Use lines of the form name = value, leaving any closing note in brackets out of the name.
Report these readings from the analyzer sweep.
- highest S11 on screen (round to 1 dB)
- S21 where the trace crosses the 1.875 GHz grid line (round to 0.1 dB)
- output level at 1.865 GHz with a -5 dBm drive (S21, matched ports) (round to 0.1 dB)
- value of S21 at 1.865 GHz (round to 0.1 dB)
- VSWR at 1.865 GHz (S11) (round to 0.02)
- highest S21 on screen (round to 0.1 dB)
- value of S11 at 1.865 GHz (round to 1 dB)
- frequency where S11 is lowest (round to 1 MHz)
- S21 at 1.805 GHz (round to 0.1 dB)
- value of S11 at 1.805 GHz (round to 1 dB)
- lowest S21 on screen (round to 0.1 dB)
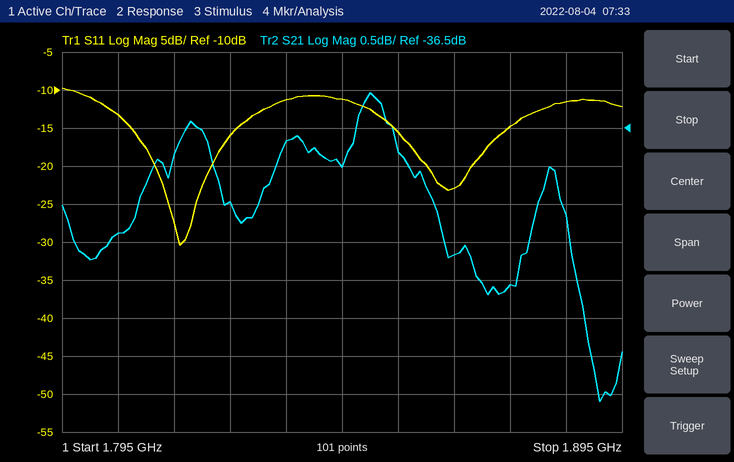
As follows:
highest S11 on screen = -10 dB
S21 where the trace crosses the 1.875 GHz grid line = -38.6 dB
output level at 1.865 GHz with a -5 dBm drive (S21, matched ports) = -43.2 dBm
value of S21 at 1.865 GHz = -38.2 dB
VSWR at 1.865 GHz (S11) = 1.16
highest S21 on screen = -36.0 dB
value of S11 at 1.865 GHz = -23 dB
frequency where S11 is lowest = 1.816 GHz
S21 at 1.805 GHz = -37.9 dB
value of S11 at 1.805 GHz = -13 dB
lowest S21 on screen = -40.1 dB
